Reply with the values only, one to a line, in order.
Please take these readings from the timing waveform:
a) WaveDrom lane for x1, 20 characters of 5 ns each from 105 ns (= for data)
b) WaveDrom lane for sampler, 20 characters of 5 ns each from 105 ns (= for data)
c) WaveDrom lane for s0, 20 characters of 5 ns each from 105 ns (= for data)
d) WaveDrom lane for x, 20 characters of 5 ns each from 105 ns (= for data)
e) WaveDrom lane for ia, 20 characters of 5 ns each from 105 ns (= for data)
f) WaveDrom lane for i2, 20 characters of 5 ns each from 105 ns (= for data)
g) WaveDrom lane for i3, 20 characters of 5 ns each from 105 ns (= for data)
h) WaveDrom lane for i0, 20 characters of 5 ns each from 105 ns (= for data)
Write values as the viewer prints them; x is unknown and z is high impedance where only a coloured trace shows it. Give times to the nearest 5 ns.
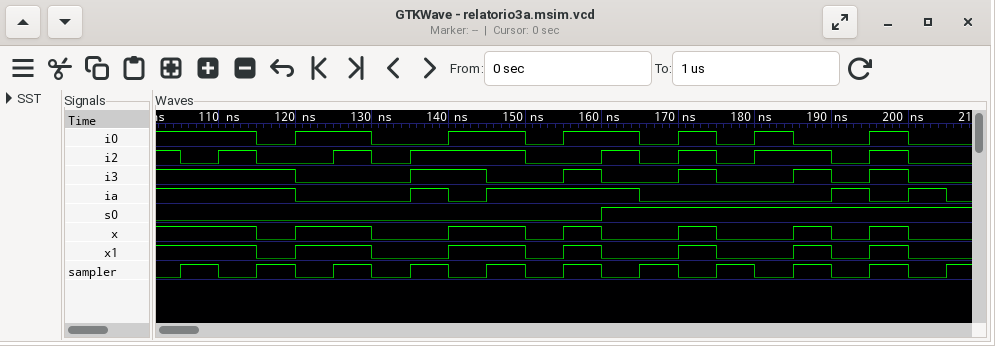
{name: 'x1', wave: '1.01.0.1.010.10.1010'}
{name: 'sampler', wave: '10101010101010101010'}
{name: 's0', wave: '0..........1........'}
{name: 'x', wave: '1.01.0.1.010.10.1010'}
{name: 'ia', wave: '1..0..101...0....101'}
{name: 'i2', wave: '010.101..0.10101.010'}
{name: 'i3', wave: '1..0..1.0.10.10.1010'}
{name: 'i0', wave: '1.01.0.1.01.01010.10'}
